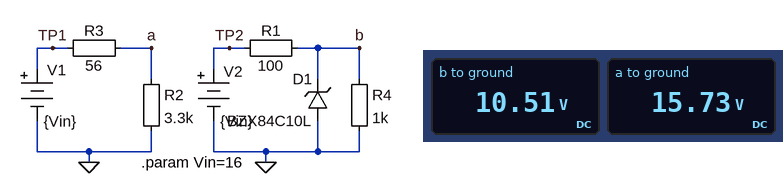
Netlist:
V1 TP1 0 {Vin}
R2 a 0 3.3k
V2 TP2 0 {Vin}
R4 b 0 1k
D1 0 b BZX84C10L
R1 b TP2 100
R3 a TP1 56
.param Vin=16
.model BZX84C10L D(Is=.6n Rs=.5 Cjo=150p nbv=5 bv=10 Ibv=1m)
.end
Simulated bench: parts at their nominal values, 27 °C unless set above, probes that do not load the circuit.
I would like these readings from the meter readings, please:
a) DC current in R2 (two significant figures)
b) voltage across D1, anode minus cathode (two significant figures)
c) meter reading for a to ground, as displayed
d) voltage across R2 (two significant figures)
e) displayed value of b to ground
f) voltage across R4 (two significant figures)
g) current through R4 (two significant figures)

4.8 mA
-11 V
15.73 V
16 V
10.51 V
11 V
11 mA
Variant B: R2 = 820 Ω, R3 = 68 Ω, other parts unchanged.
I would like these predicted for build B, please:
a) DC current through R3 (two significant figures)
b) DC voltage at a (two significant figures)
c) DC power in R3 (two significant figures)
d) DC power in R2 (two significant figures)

18 mA
15 V
22 mW
270 mW
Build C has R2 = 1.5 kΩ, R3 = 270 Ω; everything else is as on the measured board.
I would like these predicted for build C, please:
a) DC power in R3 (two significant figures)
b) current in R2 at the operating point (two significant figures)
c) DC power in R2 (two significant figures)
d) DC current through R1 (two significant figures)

22 mW
9.0 mA
120 mW
55 mA
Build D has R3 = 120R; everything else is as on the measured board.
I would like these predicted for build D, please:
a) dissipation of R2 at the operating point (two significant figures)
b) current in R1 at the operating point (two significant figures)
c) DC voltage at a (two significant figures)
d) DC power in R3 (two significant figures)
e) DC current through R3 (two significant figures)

72 mW
55 mA
15 V
2.6 mW
4.7 mA
